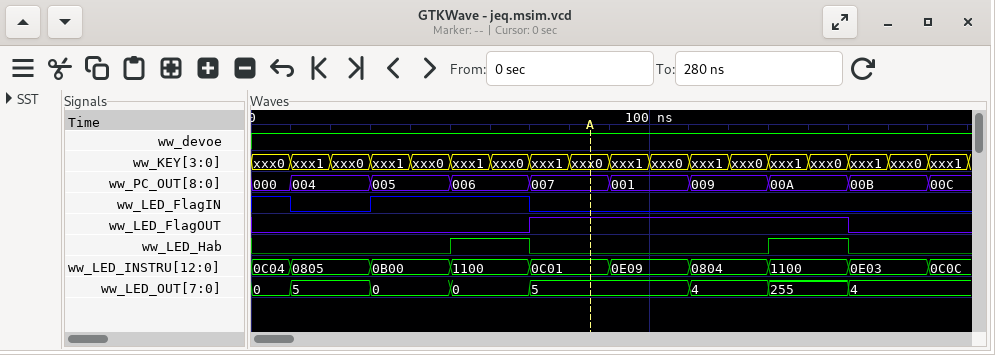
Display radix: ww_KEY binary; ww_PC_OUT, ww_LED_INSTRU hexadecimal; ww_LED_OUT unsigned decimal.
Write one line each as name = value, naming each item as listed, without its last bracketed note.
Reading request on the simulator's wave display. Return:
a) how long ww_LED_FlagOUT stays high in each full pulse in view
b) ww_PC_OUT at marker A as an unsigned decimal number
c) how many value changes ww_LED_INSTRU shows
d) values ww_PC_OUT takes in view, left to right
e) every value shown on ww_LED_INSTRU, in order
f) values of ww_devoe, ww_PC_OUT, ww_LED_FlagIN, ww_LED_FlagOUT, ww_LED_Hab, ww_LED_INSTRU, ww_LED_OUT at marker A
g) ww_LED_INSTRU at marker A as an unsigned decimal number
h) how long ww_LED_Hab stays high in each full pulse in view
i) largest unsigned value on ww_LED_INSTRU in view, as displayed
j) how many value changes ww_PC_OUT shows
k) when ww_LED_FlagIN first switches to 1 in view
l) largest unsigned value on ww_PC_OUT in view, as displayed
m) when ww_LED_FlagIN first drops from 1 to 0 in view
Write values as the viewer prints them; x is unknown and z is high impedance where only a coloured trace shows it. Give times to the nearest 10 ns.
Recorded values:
how long ww_LED_FlagOUT stays high in each full pulse in view = 80 ns
ww_PC_OUT at marker A as an unsigned decimal number = 7
how many value changes ww_LED_INSTRU shows = 9
values ww_PC_OUT takes in view, left to right = 000, 004, 005, 006, 007, 001, 009, 00A, 00B, 00C
every value shown on ww_LED_INSTRU, in order = 0C04, 0805, 0B00, 1100, 0C01, 0E09, 0804, 1100, 0E03, 0C0C
values of ww_devoe, ww_PC_OUT, ww_LED_FlagIN, ww_LED_FlagOUT, ww_LED_Hab, ww_LED_INSTRU, ww_LED_OUT at marker A = ww_devoe=1, ww_PC_OUT=007, ww_LED_FlagIN=0, ww_LED_FlagOUT=1, ww_LED_Hab=0, ww_LED_INSTRU=0C01, ww_LED_OUT=5
ww_LED_INSTRU at marker A as an unsigned decimal number = 3073
how long ww_LED_Hab stays high in each full pulse in view = 20 ns, 20 ns
largest unsigned value on ww_LED_INSTRU in view, as displayed = 1100
how many value changes ww_PC_OUT shows = 9
when ww_LED_FlagIN first switches to 1 in view = 30 ns
largest unsigned value on ww_PC_OUT in view, as displayed = 00C
when ww_LED_FlagIN first drops from 1 to 0 in view = 10 ns
